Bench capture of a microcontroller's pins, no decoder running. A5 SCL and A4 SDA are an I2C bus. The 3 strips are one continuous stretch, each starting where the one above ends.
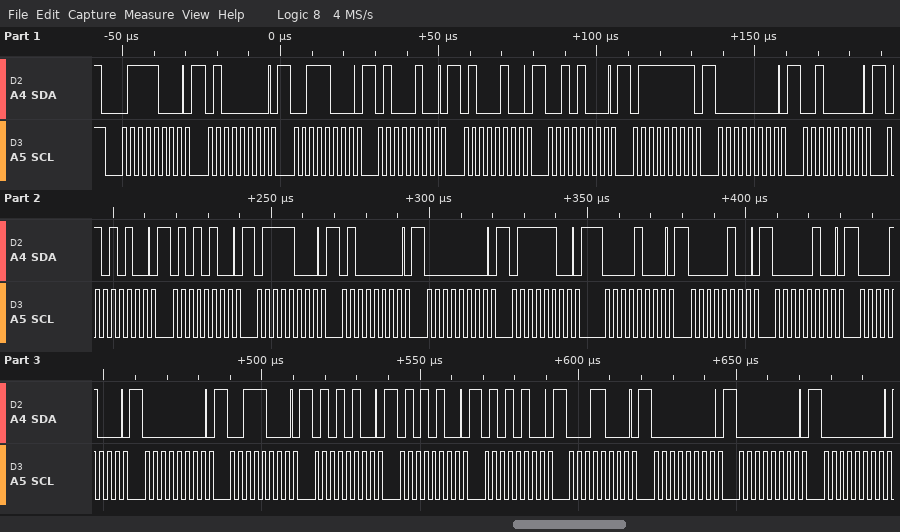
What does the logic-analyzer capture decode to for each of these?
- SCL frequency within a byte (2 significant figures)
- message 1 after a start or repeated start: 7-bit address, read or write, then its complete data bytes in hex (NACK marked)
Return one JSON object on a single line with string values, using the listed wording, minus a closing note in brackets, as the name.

{"SCL frequency within a byte": "400 kHz", "message 1 after a start or repeated start: 7-bit address, read or write, then its complete data bytes in hex": "0x3C write: 40 38 44 44 28 7F 00 20 54 54 78 40 00 7C 08 04 04 08 00 38 54 54 54 18 00 00 00"}
